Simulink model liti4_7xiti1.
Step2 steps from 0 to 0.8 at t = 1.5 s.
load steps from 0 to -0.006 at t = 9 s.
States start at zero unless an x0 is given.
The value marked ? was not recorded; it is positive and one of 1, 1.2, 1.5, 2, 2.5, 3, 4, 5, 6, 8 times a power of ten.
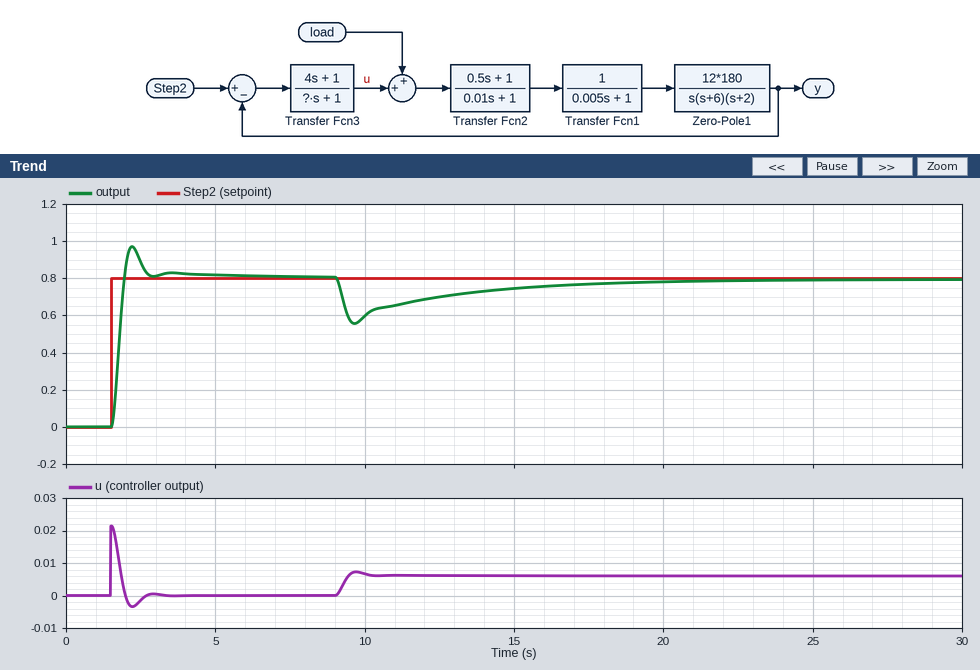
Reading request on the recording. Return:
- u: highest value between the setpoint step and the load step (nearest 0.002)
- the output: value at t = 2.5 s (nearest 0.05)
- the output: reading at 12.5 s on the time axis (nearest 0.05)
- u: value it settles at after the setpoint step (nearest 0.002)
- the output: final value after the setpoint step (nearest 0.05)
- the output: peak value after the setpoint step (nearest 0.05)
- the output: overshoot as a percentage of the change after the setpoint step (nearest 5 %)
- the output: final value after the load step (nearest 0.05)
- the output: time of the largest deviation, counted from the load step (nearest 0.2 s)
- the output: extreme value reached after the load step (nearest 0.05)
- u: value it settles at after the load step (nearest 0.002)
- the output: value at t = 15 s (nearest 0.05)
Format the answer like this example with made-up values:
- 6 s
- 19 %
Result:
- 0.022
- 0.90
- 0.70
- 0.000
- 0.80
- 0.95
- 20 %
- 0.80
- 0.6 s
- 0.55
- 0.006
- 0.75
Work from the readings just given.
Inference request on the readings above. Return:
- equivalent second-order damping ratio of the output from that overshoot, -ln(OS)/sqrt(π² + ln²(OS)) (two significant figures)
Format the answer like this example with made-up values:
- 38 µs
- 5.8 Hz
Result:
- 0.46
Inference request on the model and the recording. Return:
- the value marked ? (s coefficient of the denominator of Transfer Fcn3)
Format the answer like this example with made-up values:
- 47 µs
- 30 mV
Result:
- 150
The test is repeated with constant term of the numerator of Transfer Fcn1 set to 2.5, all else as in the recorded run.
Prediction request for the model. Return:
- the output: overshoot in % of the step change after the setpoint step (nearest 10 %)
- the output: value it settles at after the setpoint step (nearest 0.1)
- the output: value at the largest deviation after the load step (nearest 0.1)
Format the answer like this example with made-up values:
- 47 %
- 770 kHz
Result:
- 40 %
- 0.8
- 0.5
